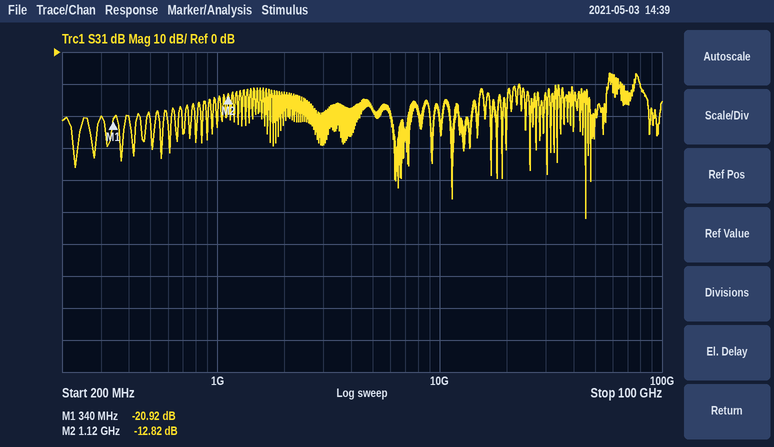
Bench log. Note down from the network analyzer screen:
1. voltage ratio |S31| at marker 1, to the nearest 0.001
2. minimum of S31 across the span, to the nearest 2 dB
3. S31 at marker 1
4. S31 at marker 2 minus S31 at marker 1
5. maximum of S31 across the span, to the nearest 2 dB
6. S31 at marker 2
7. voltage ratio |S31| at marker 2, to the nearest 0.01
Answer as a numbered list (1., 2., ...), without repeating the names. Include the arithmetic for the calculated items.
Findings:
1. 10^(-20.92/20) ≈ 0.090
2. -52 dB
3. -20.92 dB
4. -12.82 − (-20.92) = 8.10 dB
5. -6 dB
6. -12.82 dB
7. 10^(-12.82/20) ≈ 0.23
